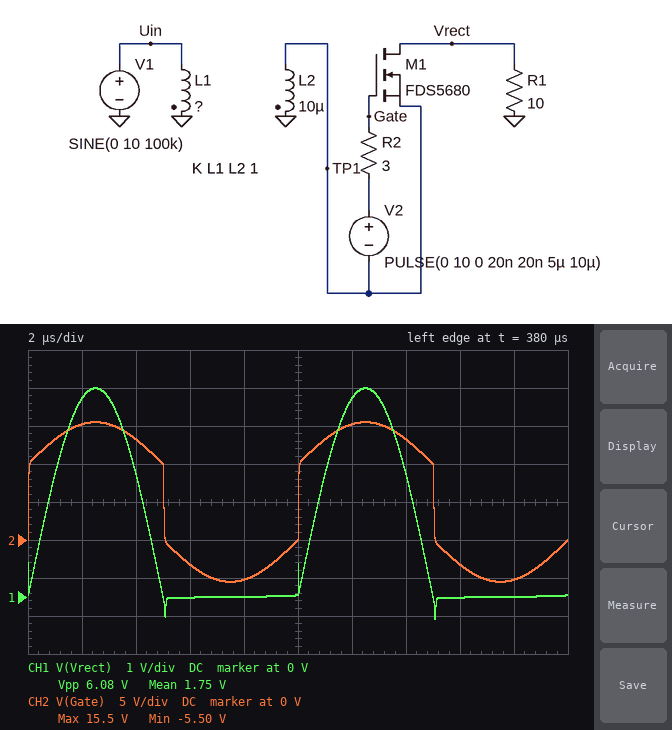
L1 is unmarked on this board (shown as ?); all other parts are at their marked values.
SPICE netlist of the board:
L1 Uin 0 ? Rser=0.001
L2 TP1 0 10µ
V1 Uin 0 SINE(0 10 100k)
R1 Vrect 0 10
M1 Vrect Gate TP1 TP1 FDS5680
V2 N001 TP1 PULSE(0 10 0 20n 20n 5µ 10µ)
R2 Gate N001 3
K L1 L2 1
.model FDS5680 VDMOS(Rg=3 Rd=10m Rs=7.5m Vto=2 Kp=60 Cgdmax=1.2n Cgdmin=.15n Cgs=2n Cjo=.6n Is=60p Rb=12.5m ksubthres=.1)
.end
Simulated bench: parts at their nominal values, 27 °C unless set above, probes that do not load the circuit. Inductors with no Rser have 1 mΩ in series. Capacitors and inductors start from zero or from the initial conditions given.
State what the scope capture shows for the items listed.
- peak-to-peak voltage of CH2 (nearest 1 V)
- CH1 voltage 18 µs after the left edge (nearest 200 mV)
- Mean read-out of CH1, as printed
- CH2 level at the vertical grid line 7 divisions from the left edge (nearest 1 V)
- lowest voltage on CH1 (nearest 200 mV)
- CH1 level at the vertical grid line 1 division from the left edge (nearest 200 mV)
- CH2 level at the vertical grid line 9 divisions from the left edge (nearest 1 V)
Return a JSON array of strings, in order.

["21 V", "0 V", "1.75 V", "13 V", "-600 mV", "5.2 V", "-5 V"]
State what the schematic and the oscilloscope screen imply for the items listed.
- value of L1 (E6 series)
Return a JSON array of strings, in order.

["33 µH"]
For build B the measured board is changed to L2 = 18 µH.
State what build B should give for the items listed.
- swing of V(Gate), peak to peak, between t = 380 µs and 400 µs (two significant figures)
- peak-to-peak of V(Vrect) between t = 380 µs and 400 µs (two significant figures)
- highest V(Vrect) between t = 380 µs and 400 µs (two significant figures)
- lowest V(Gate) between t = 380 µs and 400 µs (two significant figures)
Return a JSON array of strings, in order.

["25 V", "8.0 V", "7.4 V", "-7.4 V"]
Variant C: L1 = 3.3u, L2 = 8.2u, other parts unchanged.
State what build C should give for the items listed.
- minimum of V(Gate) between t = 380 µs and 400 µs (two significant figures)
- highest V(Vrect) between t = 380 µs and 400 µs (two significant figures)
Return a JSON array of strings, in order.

["-16 V", "16 V"]
